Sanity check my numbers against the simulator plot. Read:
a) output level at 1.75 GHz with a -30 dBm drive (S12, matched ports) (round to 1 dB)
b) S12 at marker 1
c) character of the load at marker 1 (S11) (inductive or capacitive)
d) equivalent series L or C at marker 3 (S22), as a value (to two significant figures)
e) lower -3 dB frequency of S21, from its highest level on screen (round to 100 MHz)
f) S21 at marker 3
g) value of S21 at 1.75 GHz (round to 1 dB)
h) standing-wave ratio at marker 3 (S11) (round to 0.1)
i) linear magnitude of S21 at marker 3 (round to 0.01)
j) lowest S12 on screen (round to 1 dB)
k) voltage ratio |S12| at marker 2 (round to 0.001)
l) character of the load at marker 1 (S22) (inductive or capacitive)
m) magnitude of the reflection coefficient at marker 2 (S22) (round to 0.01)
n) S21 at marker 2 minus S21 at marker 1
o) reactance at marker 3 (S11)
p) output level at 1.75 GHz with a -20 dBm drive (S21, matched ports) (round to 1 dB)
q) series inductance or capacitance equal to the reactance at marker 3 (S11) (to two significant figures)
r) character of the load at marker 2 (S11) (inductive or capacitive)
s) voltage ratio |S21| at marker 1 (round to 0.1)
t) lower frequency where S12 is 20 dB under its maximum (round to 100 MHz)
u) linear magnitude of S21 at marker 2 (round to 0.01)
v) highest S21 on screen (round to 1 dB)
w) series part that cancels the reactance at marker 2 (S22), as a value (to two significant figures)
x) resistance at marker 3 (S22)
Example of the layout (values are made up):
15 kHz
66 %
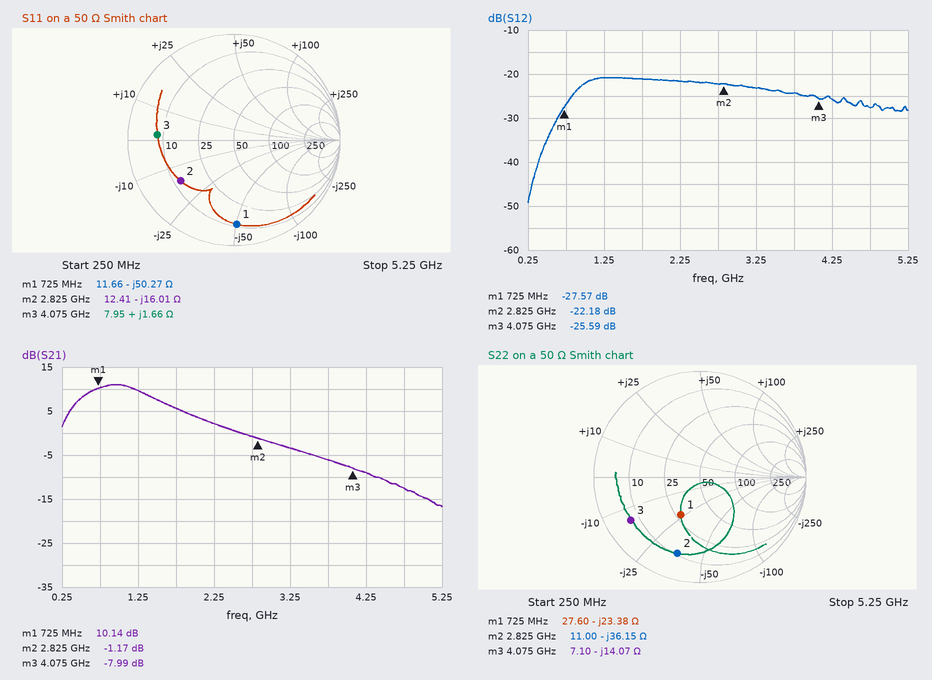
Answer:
-51 dBm
-27.57 dB
capacitive
2.8 pF
500 MHz
-7.99 dB
6 dB
6.3
0.40
-49 dB
0.078
capacitive
0.75
-11.31 dB
+1.66 Ω
-14 dBm
65 pH
capacitive
3.2
400 MHz
0.87
11 dB
2.0 nH
7.10 Ω
